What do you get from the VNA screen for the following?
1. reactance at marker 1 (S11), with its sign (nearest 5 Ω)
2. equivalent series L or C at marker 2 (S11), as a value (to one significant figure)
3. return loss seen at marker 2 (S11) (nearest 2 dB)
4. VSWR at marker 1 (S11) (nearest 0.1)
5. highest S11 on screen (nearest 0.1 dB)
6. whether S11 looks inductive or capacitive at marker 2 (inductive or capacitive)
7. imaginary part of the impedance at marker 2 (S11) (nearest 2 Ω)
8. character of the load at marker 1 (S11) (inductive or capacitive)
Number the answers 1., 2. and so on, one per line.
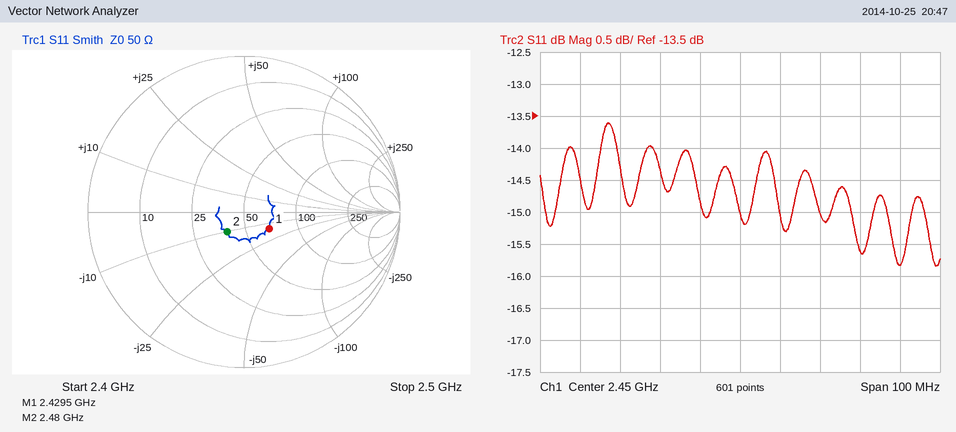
1. -15 Ω
2. 6 pF
3. 16 dB
4. 1.5
5. -13.6 dB
6. capacitive
7. -10 Ω
8. capacitive
